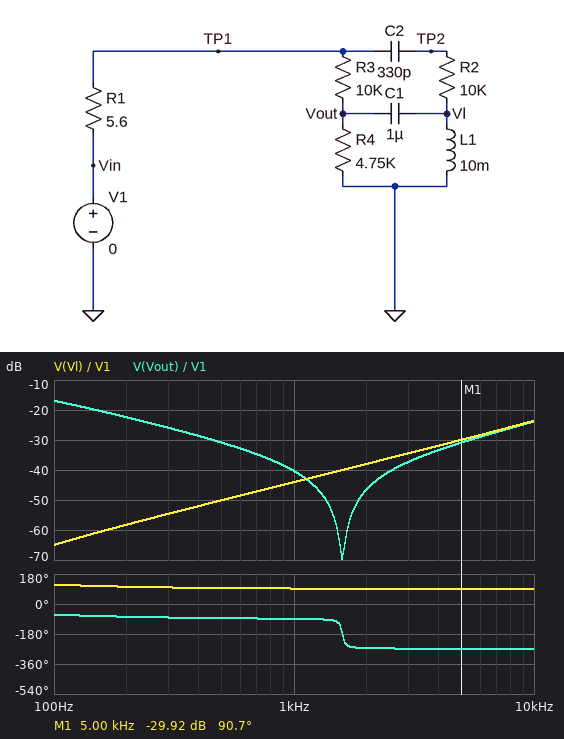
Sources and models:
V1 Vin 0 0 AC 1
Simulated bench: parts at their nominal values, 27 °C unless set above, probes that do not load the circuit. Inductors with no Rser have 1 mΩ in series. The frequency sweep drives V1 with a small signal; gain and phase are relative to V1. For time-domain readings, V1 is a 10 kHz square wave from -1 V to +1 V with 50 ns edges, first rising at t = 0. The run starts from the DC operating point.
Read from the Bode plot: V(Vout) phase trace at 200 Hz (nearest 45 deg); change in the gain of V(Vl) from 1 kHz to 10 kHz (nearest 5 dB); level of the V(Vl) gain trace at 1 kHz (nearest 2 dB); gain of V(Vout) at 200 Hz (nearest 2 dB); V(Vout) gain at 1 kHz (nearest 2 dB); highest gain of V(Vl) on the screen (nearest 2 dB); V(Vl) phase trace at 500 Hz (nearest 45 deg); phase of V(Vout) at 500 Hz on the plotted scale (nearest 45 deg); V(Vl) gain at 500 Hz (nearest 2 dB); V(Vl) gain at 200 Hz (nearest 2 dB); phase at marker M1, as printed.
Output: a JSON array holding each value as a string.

["-90 deg", "20 dB", "-44 dB", "-22 dB", "-40 dB", "-24 dB", "90 deg", "-90 deg", "-50 dB", "-58 dB", "90.7 deg"]
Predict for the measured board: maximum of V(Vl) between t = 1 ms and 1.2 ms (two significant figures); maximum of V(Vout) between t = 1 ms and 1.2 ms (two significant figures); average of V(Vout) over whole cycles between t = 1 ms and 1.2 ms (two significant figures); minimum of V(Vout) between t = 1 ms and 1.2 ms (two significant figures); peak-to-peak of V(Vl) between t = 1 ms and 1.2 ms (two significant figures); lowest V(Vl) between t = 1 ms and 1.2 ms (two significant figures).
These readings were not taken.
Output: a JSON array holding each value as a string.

["970 mV", "740 mV", "-230 mV", "-1.2 V", "1.9 V", "-970 mV"]
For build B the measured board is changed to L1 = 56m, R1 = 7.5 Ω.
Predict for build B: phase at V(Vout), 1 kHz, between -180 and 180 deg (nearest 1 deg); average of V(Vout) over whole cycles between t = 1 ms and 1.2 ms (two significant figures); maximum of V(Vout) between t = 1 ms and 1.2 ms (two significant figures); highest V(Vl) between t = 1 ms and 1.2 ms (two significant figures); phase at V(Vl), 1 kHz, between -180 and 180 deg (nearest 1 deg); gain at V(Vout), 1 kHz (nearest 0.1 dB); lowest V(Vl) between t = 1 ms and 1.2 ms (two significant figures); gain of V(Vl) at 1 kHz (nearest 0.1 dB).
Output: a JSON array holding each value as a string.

["89 deg", "-230 mV", "720 mV", "950 mV", "88 deg", "-34.3 dB", "-950 mV", "-29.1 dB"]
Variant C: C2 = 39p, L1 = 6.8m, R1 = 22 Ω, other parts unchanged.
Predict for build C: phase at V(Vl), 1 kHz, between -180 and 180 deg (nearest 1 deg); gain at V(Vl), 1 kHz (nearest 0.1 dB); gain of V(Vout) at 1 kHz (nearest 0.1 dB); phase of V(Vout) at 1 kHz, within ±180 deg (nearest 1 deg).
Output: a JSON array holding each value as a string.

["92 deg", "-47.4 dB", "-38.7 dB", "-88 deg"]
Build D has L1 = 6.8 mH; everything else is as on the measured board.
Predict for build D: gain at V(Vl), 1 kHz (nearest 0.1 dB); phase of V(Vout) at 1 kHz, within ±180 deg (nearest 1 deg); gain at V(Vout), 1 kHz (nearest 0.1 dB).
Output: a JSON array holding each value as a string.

["-47.4 dB", "-88 deg", "-38.7 dB"]
